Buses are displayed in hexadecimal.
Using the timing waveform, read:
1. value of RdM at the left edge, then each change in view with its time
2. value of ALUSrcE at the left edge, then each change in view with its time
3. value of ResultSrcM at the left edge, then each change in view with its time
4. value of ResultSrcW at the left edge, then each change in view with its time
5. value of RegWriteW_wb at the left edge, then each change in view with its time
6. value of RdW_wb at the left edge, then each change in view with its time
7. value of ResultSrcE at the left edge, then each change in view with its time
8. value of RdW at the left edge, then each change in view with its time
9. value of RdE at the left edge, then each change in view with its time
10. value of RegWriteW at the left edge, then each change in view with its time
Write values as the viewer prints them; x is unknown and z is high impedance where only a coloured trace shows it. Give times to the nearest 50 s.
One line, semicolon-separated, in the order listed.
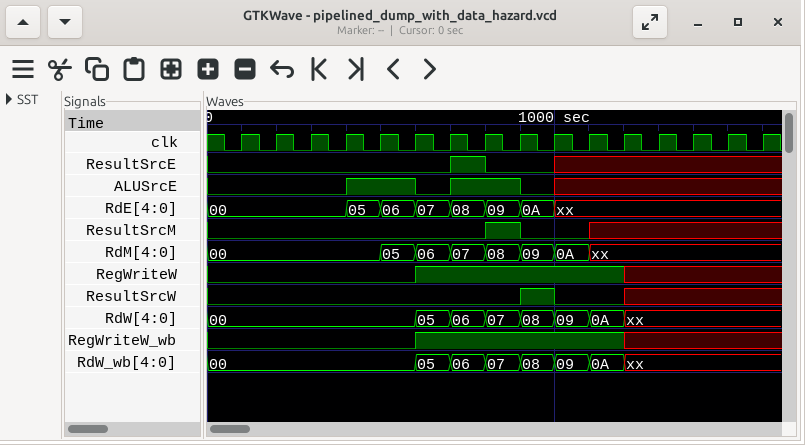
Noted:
00, 05 at 500 s, 06 at 600 s, 07 at 700 s, 08 at 800 s, 09 at 900 s, 0A at 1000 s, xx at 1100 s; 0, 1 at 400 s, 0 at 600 s, 1 at 700 s, 0 at 900 s, x at 1000 s; 0, 1 at 800 s, 0 at 900 s, x at 1100 s; 0, 1 at 900 s, 0 at 1000 s, x at 1200 s; 0, 1 at 600 s, x at 1200 s; 00, 05 at 600 s, 06 at 700 s, 07 at 800 s, 08 at 900 s, 09 at 1000 s, 0A at 1100 s, xx at 1200 s; 0, 1 at 700 s, 0 at 800 s, x at 1000 s; 00, 05 at 600 s, 06 at 700 s, 07 at 800 s, 08 at 900 s, 09 at 1000 s, 0A at 1100 s, xx at 1200 s; 00, 05 at 400 s, 06 at 500 s, 07 at 600 s, 08 at 700 s, 09 at 800 s, 0A at 900 s, xx at 1000 s; 0, 1 at 600 s, x at 1200 s
